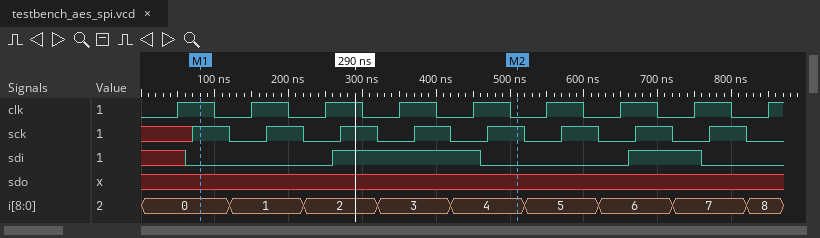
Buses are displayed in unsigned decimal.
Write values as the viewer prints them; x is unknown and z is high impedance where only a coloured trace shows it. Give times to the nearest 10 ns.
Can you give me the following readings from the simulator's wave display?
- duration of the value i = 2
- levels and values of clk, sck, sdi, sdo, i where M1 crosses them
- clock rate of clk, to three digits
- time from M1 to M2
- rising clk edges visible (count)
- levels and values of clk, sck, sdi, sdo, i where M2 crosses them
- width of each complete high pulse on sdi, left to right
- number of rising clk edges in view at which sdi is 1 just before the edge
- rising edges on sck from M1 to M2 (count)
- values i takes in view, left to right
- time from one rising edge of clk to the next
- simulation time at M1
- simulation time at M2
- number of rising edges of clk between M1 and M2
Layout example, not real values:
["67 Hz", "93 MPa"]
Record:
["100 ns", "clk=1, sck=1, sdi=0, sdo=x, i=0", "10.0 MHz", "430 ns", "9", "clk=0, sck=1, sdi=0, sdo=x, i=4", "200 ns, 100 ns", "3", "4", "0, 1, 2, 3, 4, 5, 6, 7, 8", "100 ns", "80 ns", "510 ns", "4"]
